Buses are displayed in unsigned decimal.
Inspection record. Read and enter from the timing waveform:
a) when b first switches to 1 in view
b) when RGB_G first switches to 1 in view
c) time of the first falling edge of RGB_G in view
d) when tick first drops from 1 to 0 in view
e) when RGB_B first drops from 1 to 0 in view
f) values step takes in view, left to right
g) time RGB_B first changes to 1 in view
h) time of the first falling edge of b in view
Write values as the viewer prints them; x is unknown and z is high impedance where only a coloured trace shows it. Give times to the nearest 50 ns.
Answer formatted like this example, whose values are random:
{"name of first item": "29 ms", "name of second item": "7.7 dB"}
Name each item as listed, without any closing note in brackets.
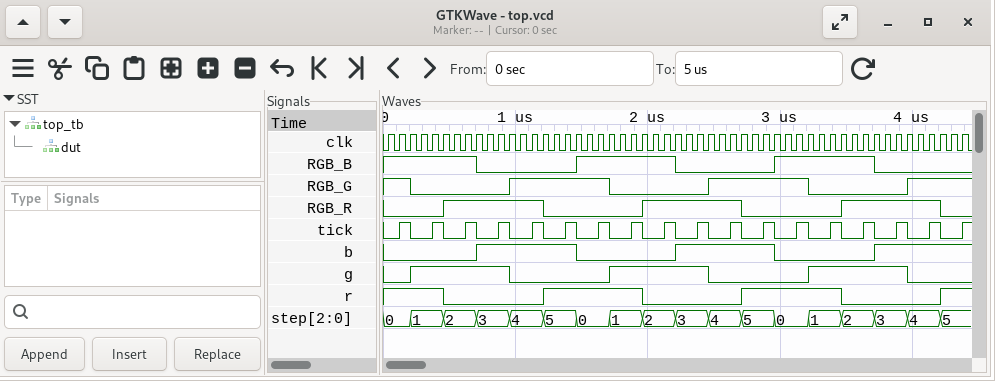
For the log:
{"when b first switches to 1 in view": "700 ns", "when RGB_G first switches to 1 in view": "950 ns", "time of the first falling edge of RGB_G in view": "200 ns", "when tick first drops from 1 to 0 in view": "200 ns", "when RGB_B first drops from 1 to 0 in view": "700 ns", "values step takes in view, left to right": "0, 1, 2, 3, 4, 5, 0, 1, 2, 3, 4, 5, 0, 1, 2, 3, 4, 5", "time RGB_B first changes to 1 in view": "1450 ns", "time of the first falling edge of b in view": "1450 ns"}
